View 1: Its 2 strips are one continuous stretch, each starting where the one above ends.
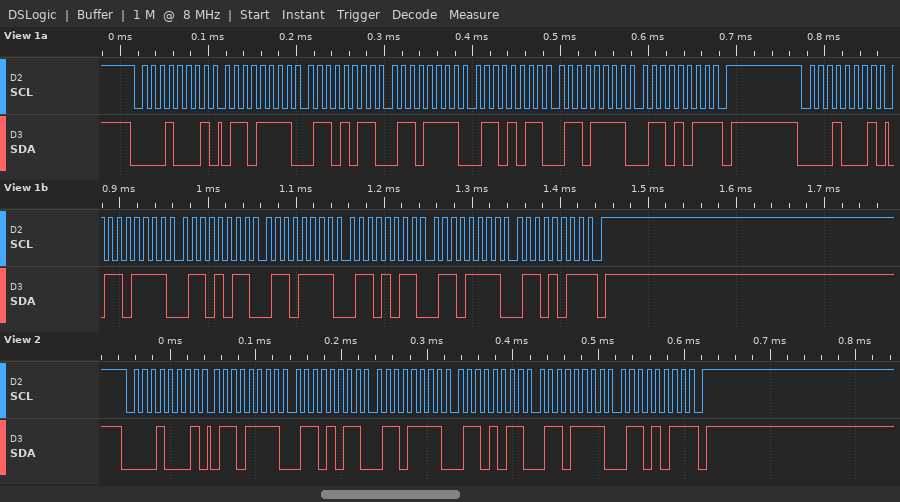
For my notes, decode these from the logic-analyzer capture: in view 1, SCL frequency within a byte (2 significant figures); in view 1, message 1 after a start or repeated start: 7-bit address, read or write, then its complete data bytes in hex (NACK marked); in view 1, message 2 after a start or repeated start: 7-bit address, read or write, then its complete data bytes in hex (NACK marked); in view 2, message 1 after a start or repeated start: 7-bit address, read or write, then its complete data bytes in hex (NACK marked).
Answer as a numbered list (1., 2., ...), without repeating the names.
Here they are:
1. 100 kHz
2. 0x08 read: 6F 6B 6F 6B 6F 6B NACK
3. 0x08 read: 6F 6B 6F 6B 6F 6B NACK
4. 0x08 read: 6F 6B 6F 6B 6F 6B NACK
